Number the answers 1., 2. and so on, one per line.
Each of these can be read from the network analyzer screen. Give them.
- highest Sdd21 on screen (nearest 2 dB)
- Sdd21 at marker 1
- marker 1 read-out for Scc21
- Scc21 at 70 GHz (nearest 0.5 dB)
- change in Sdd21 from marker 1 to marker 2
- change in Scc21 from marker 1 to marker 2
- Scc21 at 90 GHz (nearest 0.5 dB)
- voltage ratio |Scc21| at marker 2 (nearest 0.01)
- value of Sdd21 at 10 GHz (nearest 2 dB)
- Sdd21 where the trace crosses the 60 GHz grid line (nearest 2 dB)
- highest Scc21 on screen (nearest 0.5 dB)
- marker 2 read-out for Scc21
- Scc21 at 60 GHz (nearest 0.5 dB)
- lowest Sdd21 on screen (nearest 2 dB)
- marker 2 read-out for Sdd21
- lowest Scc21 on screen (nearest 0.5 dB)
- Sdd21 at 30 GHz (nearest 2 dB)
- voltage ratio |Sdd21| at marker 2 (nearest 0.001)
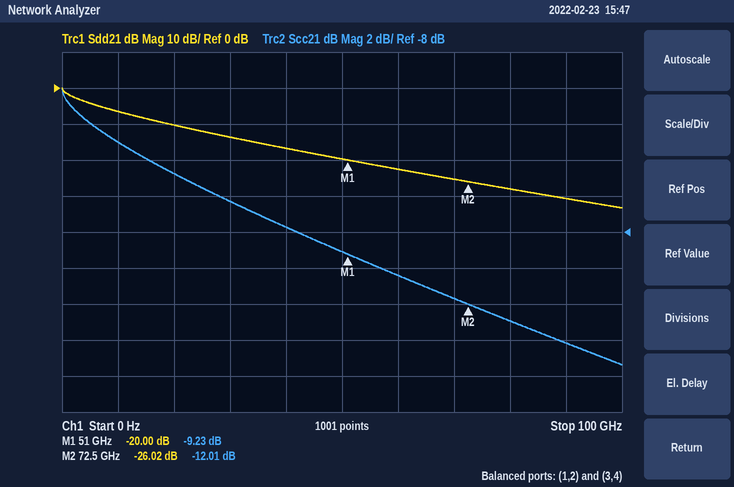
1. 0 dB
2. -20.00 dB
3. -9.23 dB
4. -11.5 dB
5. -6.02 dB
6. -2.78 dB
7. -14.0 dB
8. 0.25
9. -6 dB
10. -22 dB
11. 0.0 dB
12. -12.01 dB
13. -10.5 dB
14. -34 dB
15. -26.02 dB
16. -15.5 dB
17. -14 dB
18. 0.050
